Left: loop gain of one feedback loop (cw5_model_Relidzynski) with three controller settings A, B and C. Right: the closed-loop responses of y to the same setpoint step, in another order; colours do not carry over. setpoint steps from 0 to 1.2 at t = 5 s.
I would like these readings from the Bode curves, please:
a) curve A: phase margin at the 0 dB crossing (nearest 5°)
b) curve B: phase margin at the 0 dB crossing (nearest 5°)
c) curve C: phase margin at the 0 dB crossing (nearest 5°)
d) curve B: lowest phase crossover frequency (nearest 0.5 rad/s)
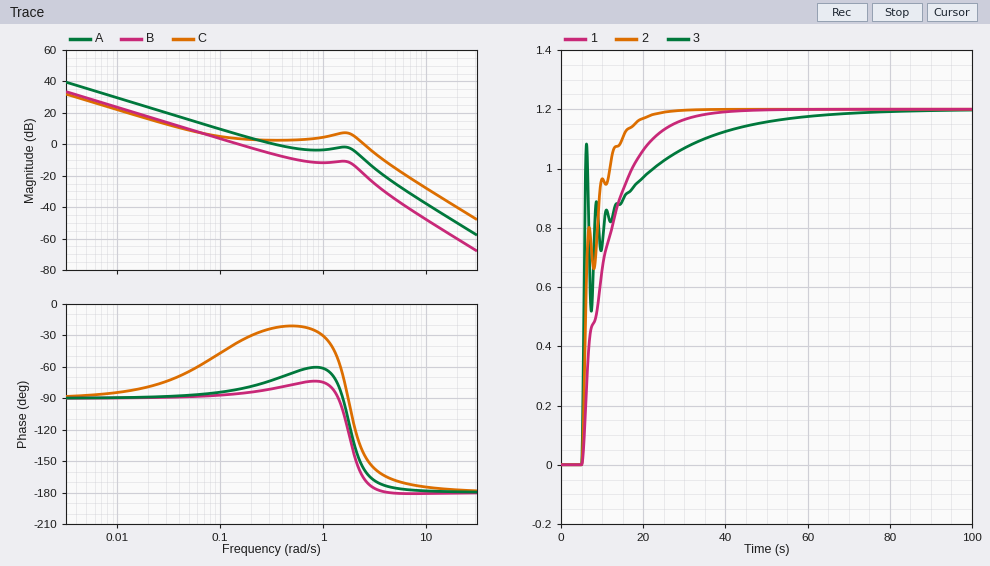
110°
95°
35°
4.5 rad/s
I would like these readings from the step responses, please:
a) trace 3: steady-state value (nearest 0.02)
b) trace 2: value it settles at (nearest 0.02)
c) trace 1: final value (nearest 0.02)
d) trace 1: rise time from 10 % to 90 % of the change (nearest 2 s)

1.20
1.20
1.20
16 s
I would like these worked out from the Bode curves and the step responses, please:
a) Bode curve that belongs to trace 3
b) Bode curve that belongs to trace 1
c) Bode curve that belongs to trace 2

C
B
A
